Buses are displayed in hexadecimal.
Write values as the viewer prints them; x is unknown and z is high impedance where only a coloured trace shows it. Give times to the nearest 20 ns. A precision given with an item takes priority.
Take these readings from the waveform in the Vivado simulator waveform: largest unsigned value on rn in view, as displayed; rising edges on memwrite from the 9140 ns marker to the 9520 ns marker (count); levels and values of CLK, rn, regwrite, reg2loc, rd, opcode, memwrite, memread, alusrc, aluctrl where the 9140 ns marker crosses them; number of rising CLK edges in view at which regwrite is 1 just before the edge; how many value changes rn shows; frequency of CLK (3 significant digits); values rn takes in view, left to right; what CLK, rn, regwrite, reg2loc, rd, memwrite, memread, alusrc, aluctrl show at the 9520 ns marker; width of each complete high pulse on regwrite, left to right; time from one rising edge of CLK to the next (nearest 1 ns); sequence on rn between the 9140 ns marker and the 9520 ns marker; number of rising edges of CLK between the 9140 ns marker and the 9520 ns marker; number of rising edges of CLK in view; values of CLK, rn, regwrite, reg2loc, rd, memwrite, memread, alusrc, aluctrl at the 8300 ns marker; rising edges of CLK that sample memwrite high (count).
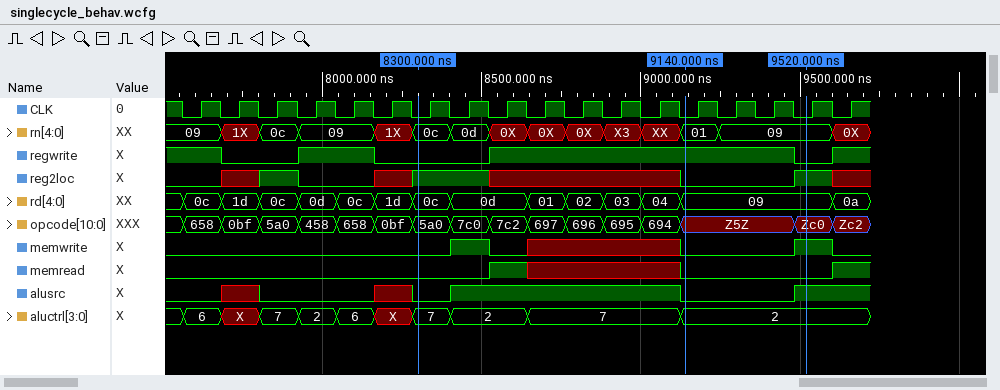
0d
1
CLK=0, rn=01, regwrite=1, reg2loc=0, rd=09, opcode=Z5Z, memwrite=0, memread=0, alusrc=0, aluctrl=2
12
14
8.33 MHz
09, 1X, 0c, 09, 1X, 0c, 0d, 0X, 0X, 0X, X3, XX, 01, 09, 0X
CLK=0, rn=09, regwrite=0, reg2loc=1, rd=09, memwrite=1, memread=0, alusrc=1, aluctrl=2
240 ns, 960 ns
120 ns
01, 09
3
18
CLK=0, rn=0c, regwrite=0, reg2loc=1, rd=0c, memwrite=0, memread=0, alusrc=0, aluctrl=7
2
